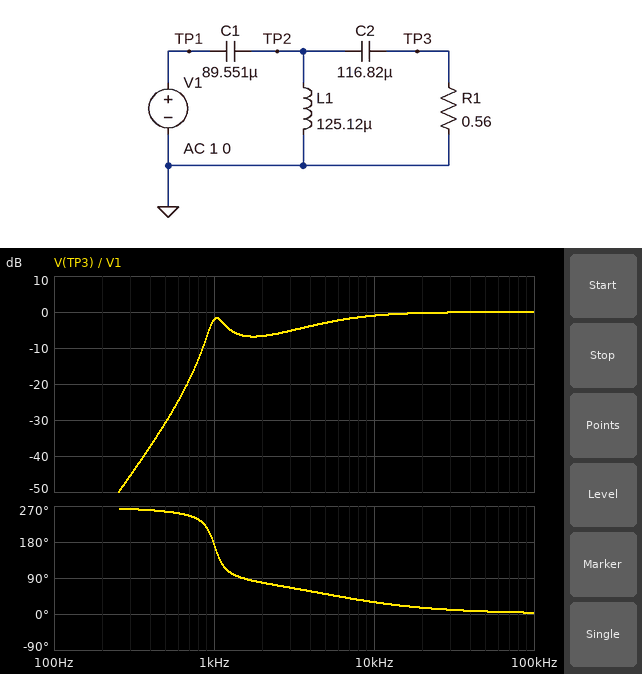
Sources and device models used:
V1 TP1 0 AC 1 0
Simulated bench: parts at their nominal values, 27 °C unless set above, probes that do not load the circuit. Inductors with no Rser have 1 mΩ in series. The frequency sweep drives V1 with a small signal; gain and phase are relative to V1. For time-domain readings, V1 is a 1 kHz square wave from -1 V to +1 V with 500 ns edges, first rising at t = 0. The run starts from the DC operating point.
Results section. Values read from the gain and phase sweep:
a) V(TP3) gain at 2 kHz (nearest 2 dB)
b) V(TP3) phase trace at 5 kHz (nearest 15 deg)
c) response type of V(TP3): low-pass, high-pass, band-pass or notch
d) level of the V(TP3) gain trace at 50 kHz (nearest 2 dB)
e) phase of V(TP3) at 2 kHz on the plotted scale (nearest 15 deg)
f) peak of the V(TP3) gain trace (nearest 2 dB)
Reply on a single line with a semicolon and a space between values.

-6 dB; 45 deg; high-pass; 0 dB; 75 deg; 0 dB
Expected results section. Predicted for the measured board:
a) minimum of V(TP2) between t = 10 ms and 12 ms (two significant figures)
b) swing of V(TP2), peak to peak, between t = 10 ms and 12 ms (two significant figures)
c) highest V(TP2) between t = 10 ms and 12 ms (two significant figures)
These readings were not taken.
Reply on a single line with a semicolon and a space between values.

-4.0 V; 8.0 V; 4.0 V
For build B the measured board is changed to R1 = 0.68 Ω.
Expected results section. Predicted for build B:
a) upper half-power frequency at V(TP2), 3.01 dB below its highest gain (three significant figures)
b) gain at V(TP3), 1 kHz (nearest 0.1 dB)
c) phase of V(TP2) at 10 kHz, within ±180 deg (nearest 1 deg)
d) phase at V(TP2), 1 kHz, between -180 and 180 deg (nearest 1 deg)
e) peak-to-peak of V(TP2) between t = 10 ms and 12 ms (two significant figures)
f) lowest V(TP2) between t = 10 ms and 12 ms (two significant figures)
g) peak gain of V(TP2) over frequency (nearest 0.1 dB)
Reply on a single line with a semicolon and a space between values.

1.25 kHz; -2.1 dB; 14 deg; 112 deg; 7.1 V; -3.5 V; 5.4 dB
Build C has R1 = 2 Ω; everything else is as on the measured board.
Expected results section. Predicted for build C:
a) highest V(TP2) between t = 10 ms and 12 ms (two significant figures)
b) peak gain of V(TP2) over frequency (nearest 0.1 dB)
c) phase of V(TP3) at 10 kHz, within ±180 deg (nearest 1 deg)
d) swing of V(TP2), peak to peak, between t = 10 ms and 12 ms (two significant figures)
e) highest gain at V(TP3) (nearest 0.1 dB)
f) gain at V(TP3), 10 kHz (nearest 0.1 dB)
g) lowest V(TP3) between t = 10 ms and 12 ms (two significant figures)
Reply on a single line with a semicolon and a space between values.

2.0 V; 5.6 dB; 9 deg; 4.0 V; 4.7 dB; 0.1 dB; -1.5 V
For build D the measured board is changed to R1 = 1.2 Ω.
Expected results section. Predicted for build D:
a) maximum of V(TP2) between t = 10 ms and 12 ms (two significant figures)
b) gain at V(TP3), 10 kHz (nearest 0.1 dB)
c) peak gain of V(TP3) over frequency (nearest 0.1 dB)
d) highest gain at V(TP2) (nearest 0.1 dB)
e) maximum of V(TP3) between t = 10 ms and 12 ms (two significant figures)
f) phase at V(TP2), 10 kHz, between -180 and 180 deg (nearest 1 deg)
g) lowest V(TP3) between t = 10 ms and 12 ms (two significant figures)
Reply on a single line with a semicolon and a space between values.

2.6 V; -0.1 dB; 0.9 dB; 3.7 dB; 1.7 V; 8 deg; -1.7 V
